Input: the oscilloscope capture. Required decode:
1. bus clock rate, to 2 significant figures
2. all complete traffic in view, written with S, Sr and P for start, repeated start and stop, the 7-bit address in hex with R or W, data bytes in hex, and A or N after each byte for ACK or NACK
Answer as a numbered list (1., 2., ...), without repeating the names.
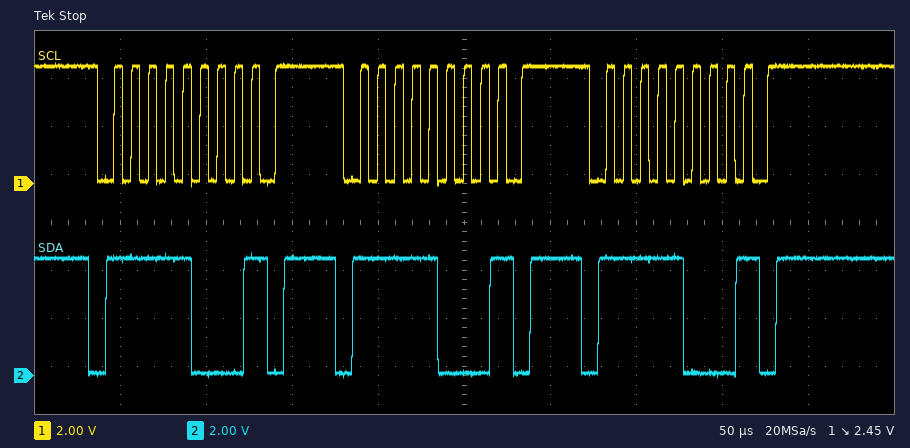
1. 100 kHz
2. S 7CW N P S 7CW N P S 7CW N P
